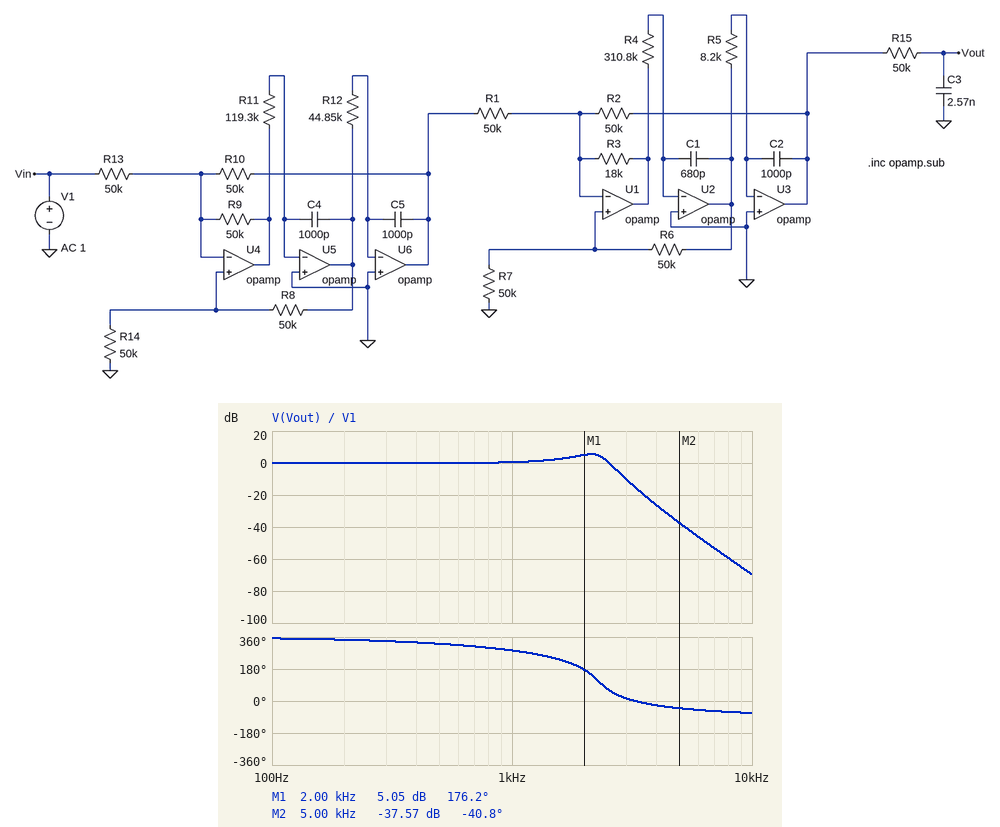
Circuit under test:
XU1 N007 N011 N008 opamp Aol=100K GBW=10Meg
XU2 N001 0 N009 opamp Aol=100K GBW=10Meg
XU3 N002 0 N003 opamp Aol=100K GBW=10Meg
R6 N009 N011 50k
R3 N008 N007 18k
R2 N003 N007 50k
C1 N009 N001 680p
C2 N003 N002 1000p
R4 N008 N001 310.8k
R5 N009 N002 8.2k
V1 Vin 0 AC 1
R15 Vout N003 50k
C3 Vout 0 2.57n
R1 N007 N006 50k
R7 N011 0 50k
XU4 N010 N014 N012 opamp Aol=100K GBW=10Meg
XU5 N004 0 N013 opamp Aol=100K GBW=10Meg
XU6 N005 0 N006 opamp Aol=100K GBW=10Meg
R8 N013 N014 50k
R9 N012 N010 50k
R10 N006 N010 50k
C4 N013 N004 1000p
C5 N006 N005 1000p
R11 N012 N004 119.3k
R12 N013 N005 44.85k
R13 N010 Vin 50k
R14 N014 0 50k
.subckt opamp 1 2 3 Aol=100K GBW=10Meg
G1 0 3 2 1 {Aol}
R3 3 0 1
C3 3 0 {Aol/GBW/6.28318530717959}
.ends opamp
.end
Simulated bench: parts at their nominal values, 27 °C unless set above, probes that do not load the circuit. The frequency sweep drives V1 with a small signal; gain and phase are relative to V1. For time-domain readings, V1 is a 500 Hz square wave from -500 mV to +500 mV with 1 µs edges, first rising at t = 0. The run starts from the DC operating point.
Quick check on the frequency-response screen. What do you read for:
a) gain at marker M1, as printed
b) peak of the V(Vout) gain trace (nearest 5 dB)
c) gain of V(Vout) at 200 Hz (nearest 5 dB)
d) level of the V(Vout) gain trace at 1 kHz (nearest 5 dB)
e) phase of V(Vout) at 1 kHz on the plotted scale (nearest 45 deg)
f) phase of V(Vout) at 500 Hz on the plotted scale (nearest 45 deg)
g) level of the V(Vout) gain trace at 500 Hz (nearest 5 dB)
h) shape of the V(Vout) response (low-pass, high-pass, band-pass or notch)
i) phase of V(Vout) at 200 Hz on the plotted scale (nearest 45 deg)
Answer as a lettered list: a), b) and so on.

a) 5.05 dB
b) 5 dB
c) 0 dB
d) 0 dB
e) 270 deg
f) 315 deg
g) 0 dB
h) low-pass
i) 360 deg
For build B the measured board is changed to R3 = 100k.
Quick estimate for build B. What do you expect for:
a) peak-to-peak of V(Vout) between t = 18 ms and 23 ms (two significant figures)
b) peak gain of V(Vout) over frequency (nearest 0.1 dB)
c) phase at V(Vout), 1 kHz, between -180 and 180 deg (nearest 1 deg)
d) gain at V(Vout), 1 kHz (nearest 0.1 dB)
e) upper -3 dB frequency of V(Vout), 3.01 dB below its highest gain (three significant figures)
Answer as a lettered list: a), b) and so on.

a) 1.0 V
b) 0 dB
c) -71 deg
d) -0.9 dB
e) 1.99 kHz
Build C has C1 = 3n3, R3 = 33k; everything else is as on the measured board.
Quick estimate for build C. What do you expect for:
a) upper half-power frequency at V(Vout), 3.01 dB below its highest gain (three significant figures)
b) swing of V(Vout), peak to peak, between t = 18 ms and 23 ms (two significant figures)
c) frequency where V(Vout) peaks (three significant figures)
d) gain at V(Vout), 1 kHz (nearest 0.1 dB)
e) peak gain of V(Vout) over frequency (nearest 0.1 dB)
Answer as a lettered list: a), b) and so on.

a) 1.49 kHz
b) 3.0 V
c) 1.40 kHz
d) 4.7 dB
e) 15.9 dB
